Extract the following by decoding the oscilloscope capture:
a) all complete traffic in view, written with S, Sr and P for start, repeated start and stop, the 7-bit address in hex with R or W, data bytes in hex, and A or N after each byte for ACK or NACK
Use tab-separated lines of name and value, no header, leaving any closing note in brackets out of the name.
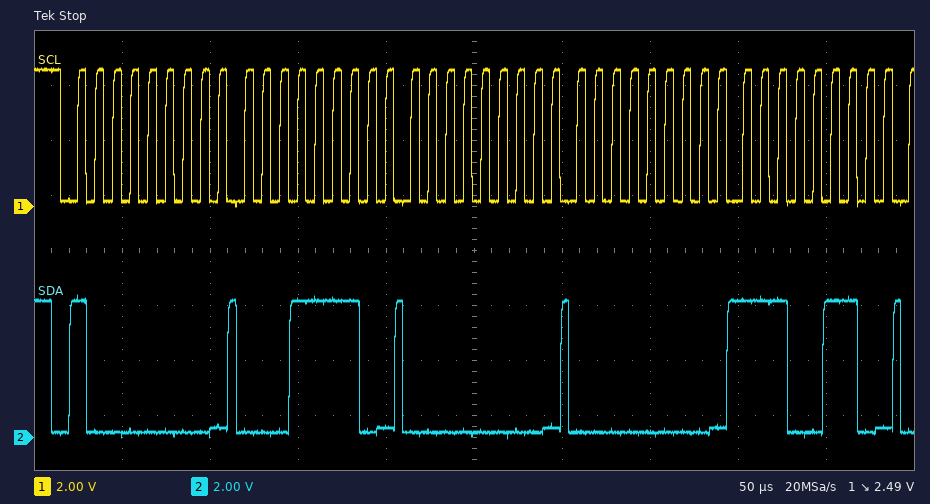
all complete traffic in view, written with S, Sr and P for start, repeated start and stop, the 7-bit address in hex with R or W, data bytes in hex, and A or N after each byte for ACK or NACK	S 40W A 1E A 00 A 00 A E6 A
